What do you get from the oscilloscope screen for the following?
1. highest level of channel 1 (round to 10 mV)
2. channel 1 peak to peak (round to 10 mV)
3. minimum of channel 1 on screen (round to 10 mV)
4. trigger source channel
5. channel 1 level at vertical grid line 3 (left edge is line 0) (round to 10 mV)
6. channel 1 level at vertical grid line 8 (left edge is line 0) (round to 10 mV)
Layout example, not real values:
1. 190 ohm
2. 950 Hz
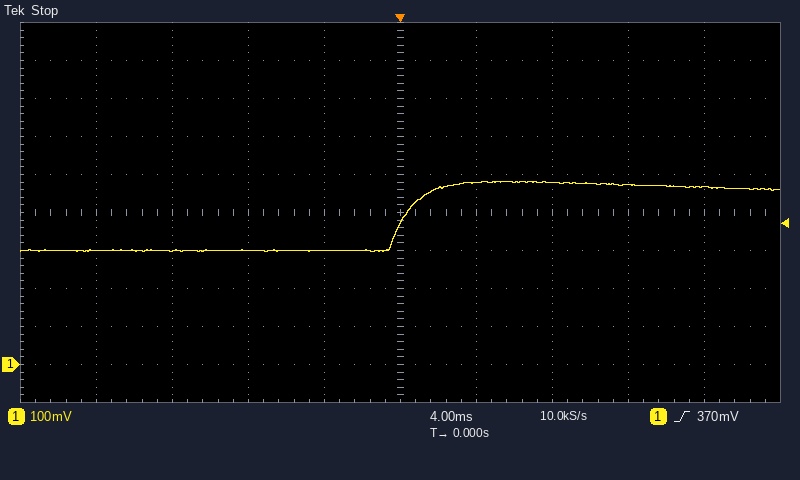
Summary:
1. 480 mV
2. 180 mV
3. 300 mV
4. channel 1
5. 300 mV
6. 470 mV
